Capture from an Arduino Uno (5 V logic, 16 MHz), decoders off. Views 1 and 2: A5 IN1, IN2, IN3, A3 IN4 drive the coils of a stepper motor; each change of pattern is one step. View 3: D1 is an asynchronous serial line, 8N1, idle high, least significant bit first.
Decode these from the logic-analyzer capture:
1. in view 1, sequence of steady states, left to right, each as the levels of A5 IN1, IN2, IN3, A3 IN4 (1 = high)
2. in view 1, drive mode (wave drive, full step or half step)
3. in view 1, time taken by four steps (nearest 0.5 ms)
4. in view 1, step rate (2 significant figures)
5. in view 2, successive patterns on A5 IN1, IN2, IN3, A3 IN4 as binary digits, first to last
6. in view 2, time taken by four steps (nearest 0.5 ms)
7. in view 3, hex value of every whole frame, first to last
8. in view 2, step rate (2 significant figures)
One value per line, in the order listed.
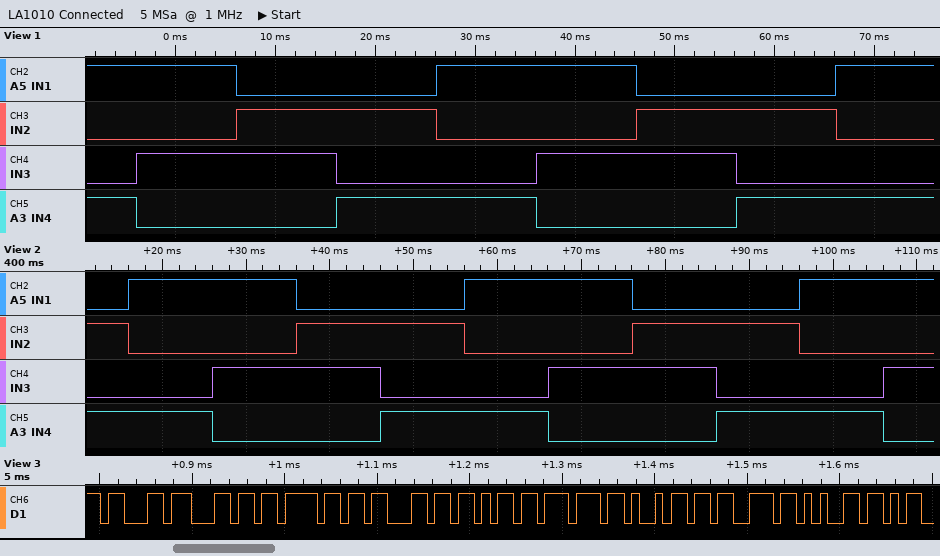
1001 1010 0110 0101 1001 1010 0110 0101 1001
full step
40.0 ms
100 steps/s
0101 1001 1010 0110 0101 1001 1010 0110 0101 1001 1010
40.0 ms
63 6C 6F 63 6B 77 69 73 65
100 steps/s
